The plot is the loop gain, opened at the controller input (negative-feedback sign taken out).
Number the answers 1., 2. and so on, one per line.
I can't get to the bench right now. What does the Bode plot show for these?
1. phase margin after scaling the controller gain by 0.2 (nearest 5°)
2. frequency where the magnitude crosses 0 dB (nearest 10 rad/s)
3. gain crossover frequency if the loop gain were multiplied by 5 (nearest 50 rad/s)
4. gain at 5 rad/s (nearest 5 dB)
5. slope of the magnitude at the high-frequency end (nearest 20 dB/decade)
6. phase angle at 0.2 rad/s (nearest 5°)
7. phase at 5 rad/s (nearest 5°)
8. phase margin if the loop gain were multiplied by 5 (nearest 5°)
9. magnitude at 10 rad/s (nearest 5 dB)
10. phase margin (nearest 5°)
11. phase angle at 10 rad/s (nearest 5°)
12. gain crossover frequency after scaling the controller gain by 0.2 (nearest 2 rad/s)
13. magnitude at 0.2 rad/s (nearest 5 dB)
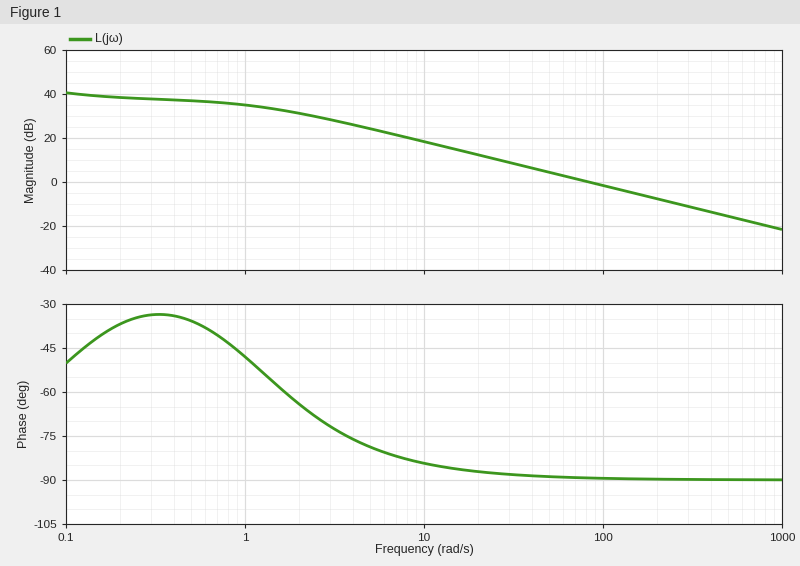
1. 95°
2. 80 rad/s
3. 400 rad/s
4. 25 dB
5. -20 dB/decade
6. -35°
7. -80°
8. 90°
9. 20 dB
10. 90°
11. -85°
12. 16 rad/s
13. 40 dB
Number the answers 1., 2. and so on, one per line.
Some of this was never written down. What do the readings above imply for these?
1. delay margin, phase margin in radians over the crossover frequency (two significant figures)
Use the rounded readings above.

1. 0.020 s
